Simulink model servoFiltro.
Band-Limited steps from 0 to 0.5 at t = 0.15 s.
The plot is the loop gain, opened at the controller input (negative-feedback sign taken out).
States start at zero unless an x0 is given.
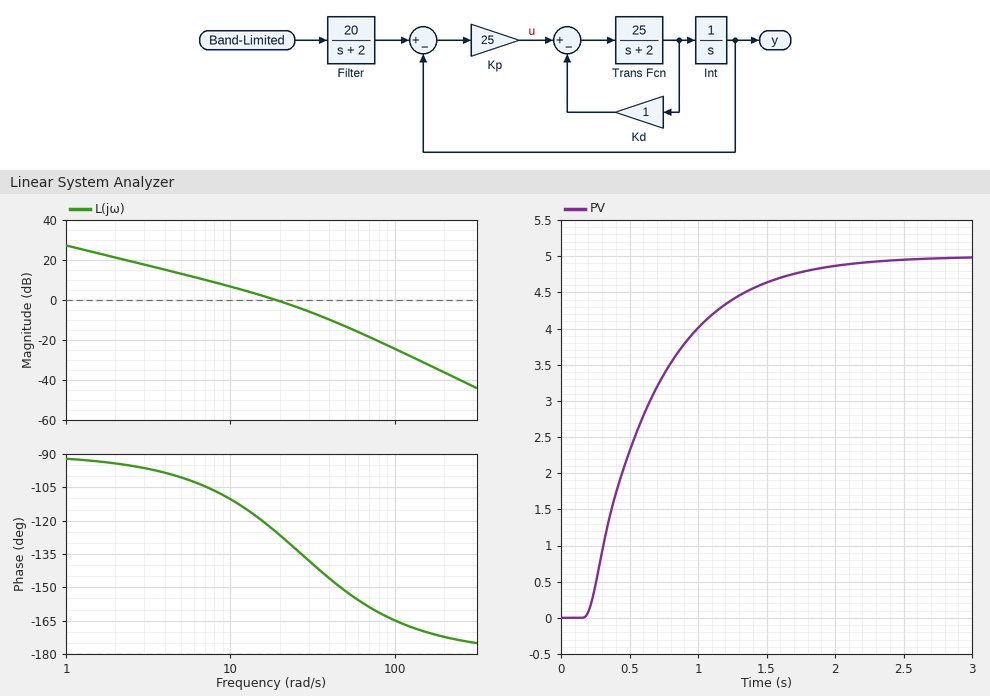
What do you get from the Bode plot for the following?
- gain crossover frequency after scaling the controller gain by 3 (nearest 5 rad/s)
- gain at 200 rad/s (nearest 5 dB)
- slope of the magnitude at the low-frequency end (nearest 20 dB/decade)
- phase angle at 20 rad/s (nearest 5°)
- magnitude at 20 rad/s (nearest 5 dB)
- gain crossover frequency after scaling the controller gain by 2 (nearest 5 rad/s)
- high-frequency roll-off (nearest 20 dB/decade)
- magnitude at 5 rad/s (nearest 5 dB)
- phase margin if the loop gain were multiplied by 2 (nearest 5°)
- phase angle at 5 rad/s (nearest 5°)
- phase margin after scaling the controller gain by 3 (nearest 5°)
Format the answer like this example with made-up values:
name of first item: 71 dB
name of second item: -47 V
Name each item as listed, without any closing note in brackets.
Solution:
gain crossover frequency after scaling the controller gain by 3: 40 rad/s
gain at 200 rad/s: -35 dB
slope of the magnitude at the low-frequency end: -20 dB/decade
phase angle at 20 rad/s: -125°
magnitude at 20 rad/s: 0 dB
gain crossover frequency after scaling the controller gain by 2: 30 rad/s
high-frequency roll-off: -40 dB/decade
magnitude at 5 rad/s: 15 dB
phase margin if the loop gain were multiplied by 2: 40°
phase angle at 5 rad/s: -100°
phase margin after scaling the controller gain by 3: 35°
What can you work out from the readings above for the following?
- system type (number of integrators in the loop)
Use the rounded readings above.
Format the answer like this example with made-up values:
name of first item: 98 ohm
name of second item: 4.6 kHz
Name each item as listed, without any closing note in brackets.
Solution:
system type: 1
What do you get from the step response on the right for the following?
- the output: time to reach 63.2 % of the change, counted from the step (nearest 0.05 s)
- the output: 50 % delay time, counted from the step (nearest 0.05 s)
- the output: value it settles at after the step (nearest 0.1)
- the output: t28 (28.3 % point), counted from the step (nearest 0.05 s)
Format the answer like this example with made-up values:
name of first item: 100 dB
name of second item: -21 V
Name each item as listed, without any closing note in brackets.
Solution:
the output: time to reach 63.2 % of the change, counted from the step: 0.55 s
the output: 50 % delay time, counted from the step: 0.40 s
the output: value it settles at after the step: 5.0
the output: t28 (28.3 % point), counted from the step: 0.20 s
